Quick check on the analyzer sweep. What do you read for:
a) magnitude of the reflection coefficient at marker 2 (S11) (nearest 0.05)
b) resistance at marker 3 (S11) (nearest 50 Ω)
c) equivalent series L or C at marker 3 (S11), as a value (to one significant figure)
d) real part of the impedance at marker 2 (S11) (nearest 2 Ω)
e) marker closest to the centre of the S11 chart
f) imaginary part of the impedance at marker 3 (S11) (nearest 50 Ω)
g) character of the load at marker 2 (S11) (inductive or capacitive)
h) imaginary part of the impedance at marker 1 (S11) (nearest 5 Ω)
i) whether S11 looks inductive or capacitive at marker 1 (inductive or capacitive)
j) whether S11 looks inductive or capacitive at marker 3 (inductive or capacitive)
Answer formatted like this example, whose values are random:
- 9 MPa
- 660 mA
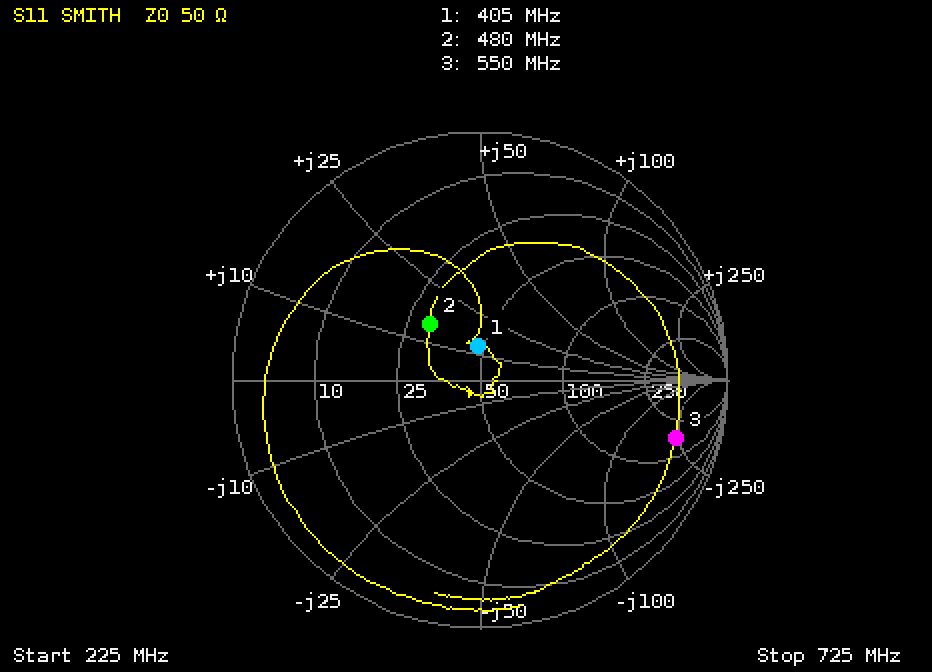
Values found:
- 0.30
- 150 Ω
- 1 pF
- 30 Ω
- marker 1
- -250 Ω
- inductive
- +15 Ω
- inductive
- capacitive
